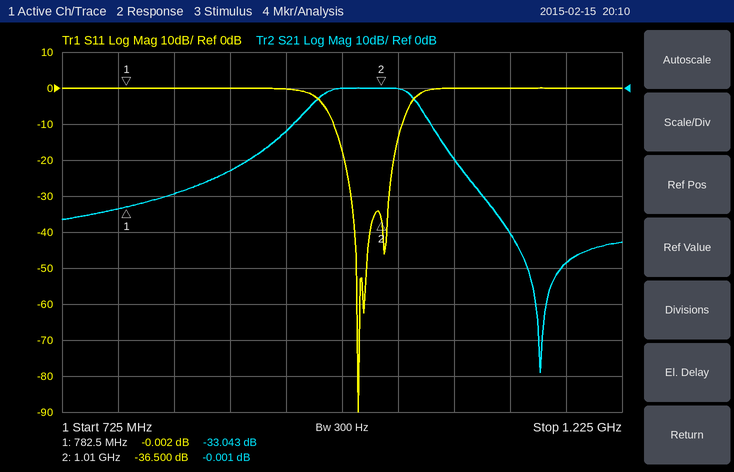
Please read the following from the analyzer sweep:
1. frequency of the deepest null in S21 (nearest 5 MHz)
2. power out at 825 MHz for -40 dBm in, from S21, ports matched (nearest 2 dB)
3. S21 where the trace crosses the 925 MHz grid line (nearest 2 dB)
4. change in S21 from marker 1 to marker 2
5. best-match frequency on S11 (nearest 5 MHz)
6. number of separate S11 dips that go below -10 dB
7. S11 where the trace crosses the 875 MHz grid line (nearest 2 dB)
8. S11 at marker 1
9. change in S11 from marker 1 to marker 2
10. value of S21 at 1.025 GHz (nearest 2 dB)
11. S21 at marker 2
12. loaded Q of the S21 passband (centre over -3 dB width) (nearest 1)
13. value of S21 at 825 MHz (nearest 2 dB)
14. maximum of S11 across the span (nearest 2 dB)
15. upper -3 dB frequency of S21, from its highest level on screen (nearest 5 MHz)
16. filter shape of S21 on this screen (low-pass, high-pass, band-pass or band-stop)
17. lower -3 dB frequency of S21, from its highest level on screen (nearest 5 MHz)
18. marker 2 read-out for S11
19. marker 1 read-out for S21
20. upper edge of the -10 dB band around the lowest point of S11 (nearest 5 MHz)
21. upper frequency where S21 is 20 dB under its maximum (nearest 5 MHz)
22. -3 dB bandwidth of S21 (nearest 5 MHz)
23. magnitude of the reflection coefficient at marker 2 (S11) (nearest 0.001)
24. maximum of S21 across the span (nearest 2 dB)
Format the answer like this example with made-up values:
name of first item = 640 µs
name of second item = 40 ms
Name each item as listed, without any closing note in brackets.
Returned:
frequency of the deepest null in S21 = 1.150 GHz
power out at 825 MHz for -40 dBm in, from S21, ports matched = -70 dBm
S21 where the trace crosses the 925 MHz grid line = -12 dB
change in S21 from marker 1 to marker 2 = 33.042 dB
best-match frequency on S11 = 990 MHz
number of separate S11 dips that go below -10 dB = 3
S11 where the trace crosses the 875 MHz grid line = 0 dB
S11 at marker 1 = -0.002 dB
change in S11 from marker 1 to marker 2 = -36.498 dB
value of S21 at 1.025 GHz = 0 dB
S21 at marker 2 = -0.001 dB
loaded Q of the S21 passband (centre over -3 dB width) = 12
value of S21 at 825 MHz = -30 dB
maximum of S11 across the span = 0 dB
upper -3 dB frequency of S21, from its highest level on screen = 1.040 GHz
filter shape of S21 on this screen = band-pass
lower -3 dB frequency of S21, from its highest level on screen = 955 MHz
marker 2 read-out for S11 = -36.500 dB
marker 1 read-out for S21 = -33.043 dB
upper edge of the -10 dB band around the lowest point of S11 = 1.030 GHz
upper frequency where S21 is 20 dB under its maximum = 1.075 GHz
-3 dB bandwidth of S21 = 85 MHz
magnitude of the reflection coefficient at marker 2 (S11) = 0.015
maximum of S21 across the span = 0 dB
